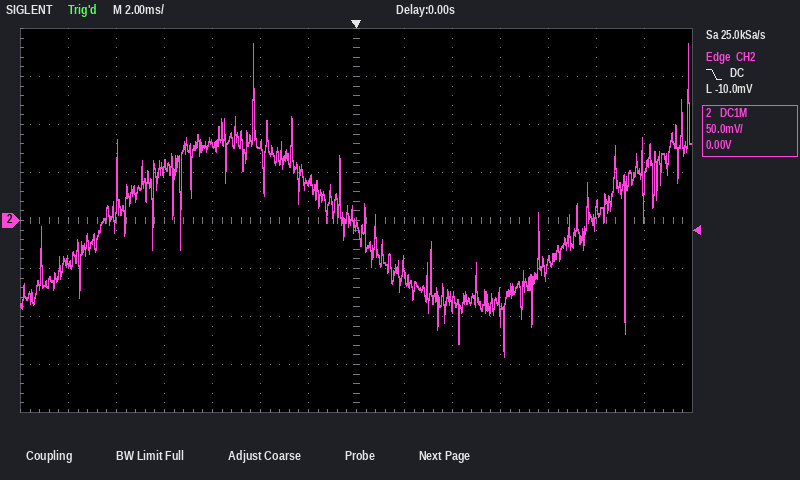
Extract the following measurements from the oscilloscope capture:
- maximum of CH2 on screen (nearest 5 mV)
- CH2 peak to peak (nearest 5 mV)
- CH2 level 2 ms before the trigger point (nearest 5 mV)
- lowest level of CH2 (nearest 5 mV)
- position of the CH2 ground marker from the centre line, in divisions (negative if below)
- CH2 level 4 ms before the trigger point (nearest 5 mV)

185 mV
325 mV
40 mV
-140 mV
0.0 div
80 mV
